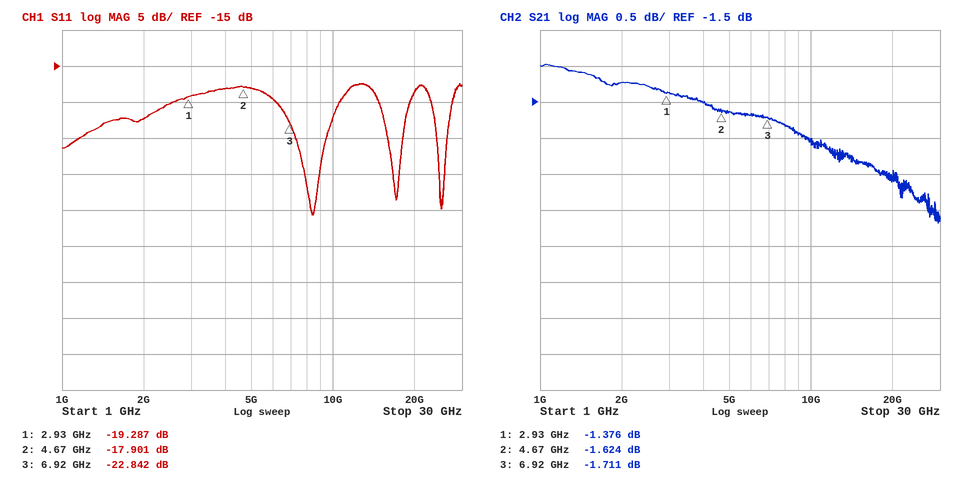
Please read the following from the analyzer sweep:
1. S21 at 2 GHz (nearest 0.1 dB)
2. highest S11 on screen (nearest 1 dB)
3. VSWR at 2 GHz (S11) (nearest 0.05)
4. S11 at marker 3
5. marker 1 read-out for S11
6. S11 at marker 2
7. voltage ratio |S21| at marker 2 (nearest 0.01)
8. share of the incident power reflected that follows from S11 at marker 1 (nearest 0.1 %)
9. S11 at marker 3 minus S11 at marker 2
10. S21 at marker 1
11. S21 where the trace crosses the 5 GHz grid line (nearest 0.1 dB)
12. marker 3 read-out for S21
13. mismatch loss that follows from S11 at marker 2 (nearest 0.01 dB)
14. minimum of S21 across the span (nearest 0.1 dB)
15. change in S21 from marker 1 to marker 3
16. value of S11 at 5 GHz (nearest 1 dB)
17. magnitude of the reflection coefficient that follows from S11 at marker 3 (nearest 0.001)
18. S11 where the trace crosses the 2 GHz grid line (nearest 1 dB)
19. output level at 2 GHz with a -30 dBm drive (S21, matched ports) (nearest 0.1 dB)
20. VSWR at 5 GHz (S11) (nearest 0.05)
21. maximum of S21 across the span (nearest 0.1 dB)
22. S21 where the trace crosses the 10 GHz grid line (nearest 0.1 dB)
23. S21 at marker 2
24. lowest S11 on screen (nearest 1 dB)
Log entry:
-1.2 dB
-17 dB
1.15
-22.842 dB
-19.287 dB
-17.901 dB
0.83
1.2 %
-4.941 dB
-1.376 dB
-1.6 dB
-1.711 dB
0.07 dB
-3.2 dB
-0.335 dB
-18 dB
0.072
-22 dB
-31.2 dBm
1.30
-1.0 dB
-2.0 dB
-1.624 dB
-36 dB
